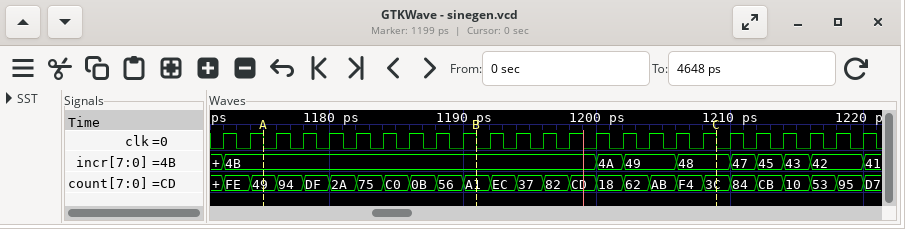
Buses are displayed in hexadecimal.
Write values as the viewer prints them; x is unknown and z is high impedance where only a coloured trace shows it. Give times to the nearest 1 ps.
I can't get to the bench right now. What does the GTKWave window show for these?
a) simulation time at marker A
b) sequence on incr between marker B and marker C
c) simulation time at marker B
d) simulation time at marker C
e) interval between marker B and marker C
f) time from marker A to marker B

1175 ps
4B, 4A, 49, 48
1191 ps
1209 ps
18 ps
16 ps
